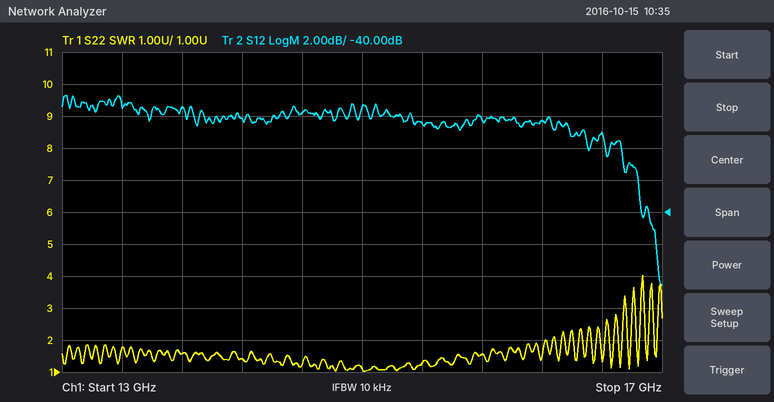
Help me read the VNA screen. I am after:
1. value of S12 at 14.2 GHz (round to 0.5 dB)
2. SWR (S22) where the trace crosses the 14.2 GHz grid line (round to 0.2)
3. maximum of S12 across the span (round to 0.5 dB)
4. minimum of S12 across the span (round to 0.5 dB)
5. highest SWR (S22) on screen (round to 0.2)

-34.0 dB
1.4
-32.5 dB
-44.5 dB
4.0
